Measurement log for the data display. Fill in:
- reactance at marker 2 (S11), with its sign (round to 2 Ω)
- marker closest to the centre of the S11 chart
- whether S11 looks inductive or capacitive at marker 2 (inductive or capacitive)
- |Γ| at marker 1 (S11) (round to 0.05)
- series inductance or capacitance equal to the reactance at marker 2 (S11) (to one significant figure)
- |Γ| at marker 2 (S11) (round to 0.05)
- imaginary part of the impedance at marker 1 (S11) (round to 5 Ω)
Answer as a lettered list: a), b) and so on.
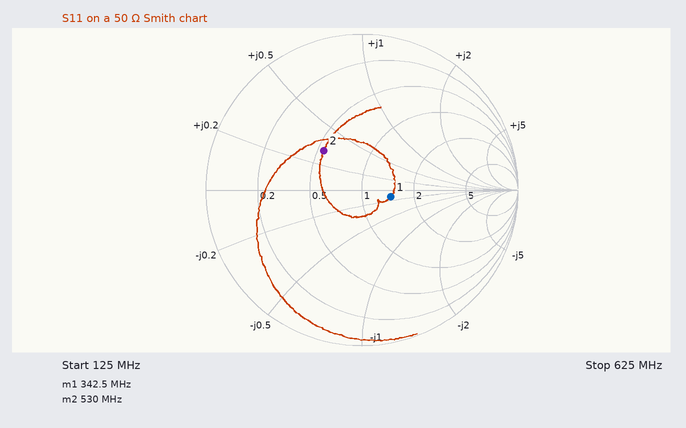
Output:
a) +16 Ω
b) marker 1
c) inductive
d) 0.20
e) 5 nH
f) 0.35
g) -5 Ω
